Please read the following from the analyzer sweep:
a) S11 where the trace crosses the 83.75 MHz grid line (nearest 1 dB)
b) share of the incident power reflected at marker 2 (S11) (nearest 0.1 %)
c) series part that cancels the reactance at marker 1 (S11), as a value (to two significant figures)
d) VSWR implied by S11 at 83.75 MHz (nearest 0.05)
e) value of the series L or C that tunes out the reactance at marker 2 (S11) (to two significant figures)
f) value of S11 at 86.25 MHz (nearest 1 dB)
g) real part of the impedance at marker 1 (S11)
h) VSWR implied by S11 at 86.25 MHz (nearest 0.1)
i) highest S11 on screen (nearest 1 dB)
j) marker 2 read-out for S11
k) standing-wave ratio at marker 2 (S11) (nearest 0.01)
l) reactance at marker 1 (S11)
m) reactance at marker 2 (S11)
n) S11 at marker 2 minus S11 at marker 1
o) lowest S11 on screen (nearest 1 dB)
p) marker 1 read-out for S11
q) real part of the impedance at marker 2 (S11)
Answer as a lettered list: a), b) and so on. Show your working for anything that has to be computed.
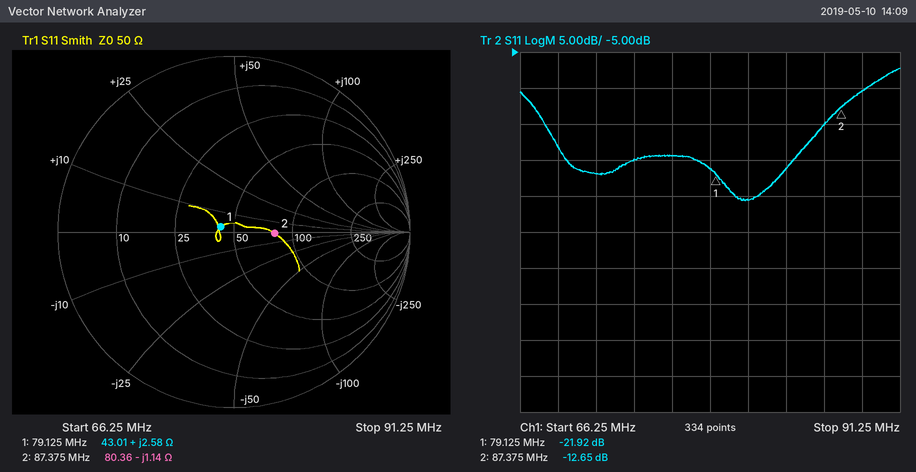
a) -21 dB
b) 10^(-12.65/10) ≈ 5.4 %
c) C = 1/(2π × 79.125 MHz × 2.58 Ω) ≈ 780 pF
d) |Γ| = 10^(-21/20) = 0.0891; VSWR = (1 + 0.0891)/(1 − 0.0891) ≈ 1.20
e) L = 1.14 Ω/(2π × 87.375 MHz) ≈ 2.1 nH
f) -15 dB
g) 43.01 Ω
h) |Γ| = 10^(-15/20) = 0.1778; VSWR = (1 + 0.1778)/(1 − 0.1778) ≈ 1.4
i) -7 dB
j) -12.65 dB
k) 1.61
l) +2.58 Ω
m) -1.14 Ω
n) -12.65 − (-21.92) = 9.27 dB
o) -26 dB
p) -21.92 dB
q) 80.36 Ω
